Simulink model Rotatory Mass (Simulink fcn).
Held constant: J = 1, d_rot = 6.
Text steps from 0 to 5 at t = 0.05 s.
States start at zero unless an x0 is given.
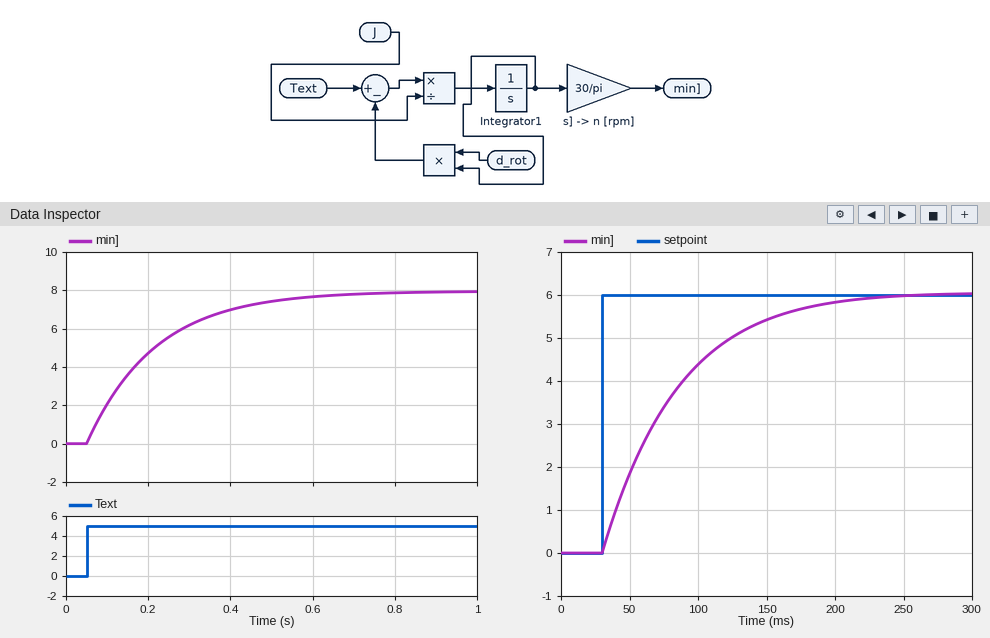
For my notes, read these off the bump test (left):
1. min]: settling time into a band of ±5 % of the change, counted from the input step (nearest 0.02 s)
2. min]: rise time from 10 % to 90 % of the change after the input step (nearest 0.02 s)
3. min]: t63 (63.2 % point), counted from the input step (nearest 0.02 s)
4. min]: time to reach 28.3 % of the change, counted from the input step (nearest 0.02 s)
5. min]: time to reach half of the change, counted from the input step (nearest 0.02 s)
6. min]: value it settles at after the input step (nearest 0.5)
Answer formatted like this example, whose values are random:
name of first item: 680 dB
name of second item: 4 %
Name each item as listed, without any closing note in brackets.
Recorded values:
min]: settling time into a band of ±5 % of the change, counted from the input step: 0.50 s
min]: rise time from 10 % to 90 % of the change after the input step: 0.36 s
min]: t63 (63.2 % point), counted from the input step: 0.16 s
min]: time to reach 28.3 % of the change, counted from the input step: 0.06 s
min]: time to reach half of the change, counted from the input step: 0.12 s
min]: value it settles at after the input step: 8.0
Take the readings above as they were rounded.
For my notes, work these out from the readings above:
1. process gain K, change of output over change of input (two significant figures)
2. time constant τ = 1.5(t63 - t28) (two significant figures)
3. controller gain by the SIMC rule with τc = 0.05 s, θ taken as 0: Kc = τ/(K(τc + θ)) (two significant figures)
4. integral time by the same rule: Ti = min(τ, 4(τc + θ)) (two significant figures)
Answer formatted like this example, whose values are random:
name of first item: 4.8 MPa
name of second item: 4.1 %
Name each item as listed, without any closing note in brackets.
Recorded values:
process gain K, change of output over change of input: 1.6
time constant τ = 1.5(t63 - t28): 0.15 s
controller gain by the SIMC rule with τc = 0.05 s, θ taken as 0: Kc = τ/(K(τc + θ)): 1.9
integral time by the same rule: Ti = min(τ, 4(τc + θ)): 0.15 s
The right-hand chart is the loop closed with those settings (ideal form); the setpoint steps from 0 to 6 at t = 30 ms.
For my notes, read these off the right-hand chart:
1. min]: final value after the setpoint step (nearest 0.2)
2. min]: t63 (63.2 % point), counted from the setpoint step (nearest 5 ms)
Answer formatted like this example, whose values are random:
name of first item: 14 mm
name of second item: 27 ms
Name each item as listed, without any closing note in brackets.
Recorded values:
min]: final value after the setpoint step: 6.0
min]: t63 (63.2 % point), counted from the setpoint step: 55 ms
